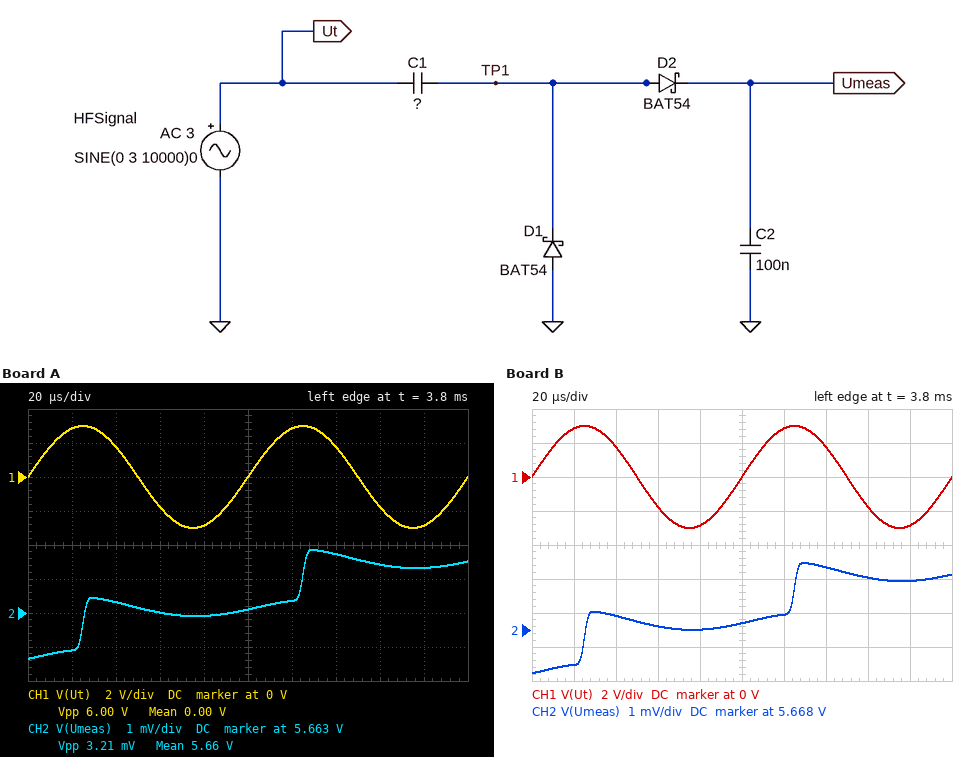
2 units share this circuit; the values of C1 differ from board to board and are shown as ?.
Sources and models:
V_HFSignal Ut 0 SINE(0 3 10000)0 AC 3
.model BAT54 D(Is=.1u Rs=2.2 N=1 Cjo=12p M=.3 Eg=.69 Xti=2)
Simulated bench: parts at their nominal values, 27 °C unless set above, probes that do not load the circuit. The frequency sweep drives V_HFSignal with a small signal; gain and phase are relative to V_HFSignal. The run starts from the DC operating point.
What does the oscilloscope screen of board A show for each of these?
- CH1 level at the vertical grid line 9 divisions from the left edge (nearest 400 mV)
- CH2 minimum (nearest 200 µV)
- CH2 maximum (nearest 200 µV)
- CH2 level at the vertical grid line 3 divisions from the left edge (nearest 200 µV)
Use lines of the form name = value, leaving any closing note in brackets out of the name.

CH1 level at the vertical grid line 9 divisions from the left edge = -2.8 V
CH2 minimum = 5.6616 V
CH2 maximum = 5.6648 V
CH2 level at the vertical grid line 3 divisions from the left edge = 5.6630 V
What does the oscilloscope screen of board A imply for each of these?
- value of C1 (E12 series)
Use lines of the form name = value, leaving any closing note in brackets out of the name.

value of C1 = 330 nF
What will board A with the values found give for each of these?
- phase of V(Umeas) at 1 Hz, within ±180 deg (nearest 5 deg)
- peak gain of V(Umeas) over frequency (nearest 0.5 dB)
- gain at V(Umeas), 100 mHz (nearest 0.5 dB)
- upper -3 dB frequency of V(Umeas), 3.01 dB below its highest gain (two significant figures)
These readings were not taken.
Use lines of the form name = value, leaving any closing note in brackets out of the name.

phase of V(Umeas) at 1 Hz, within ±180 deg = 45 deg
peak gain of V(Umeas) over frequency = -4.0 dB
gain at V(Umeas), 100 mHz = -25.5 dB
upper -3 dB frequency of V(Umeas), 3.01 dB below its highest gain = 11 Hz
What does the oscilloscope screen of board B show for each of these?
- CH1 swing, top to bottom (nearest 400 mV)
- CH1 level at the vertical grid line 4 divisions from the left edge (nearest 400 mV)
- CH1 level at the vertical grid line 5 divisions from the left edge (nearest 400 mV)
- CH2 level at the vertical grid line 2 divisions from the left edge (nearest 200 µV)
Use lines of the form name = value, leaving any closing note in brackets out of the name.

CH1 swing, top to bottom = 6.0 V
CH1 level at the vertical grid line 4 divisions from the left edge = -2.8 V
CH1 level at the vertical grid line 5 divisions from the left edge = 0 V
CH2 level at the vertical grid line 2 divisions from the left edge = 5.6684 V
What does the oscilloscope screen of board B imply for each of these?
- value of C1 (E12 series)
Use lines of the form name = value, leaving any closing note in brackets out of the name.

value of C1 = 220 nF
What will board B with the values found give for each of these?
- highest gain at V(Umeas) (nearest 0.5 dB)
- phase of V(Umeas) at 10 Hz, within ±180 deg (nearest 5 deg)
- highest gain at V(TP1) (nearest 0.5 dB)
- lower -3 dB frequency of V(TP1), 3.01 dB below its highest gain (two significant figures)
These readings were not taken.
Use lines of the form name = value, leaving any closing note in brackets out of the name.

highest gain at V(Umeas) = -5.5 dB
phase of V(Umeas) at 10 Hz, within ±180 deg = -35 deg
highest gain at V(TP1) = 0 dB
lower -3 dB frequency of V(TP1), 3.01 dB below its highest gain = 6.0 Hz
